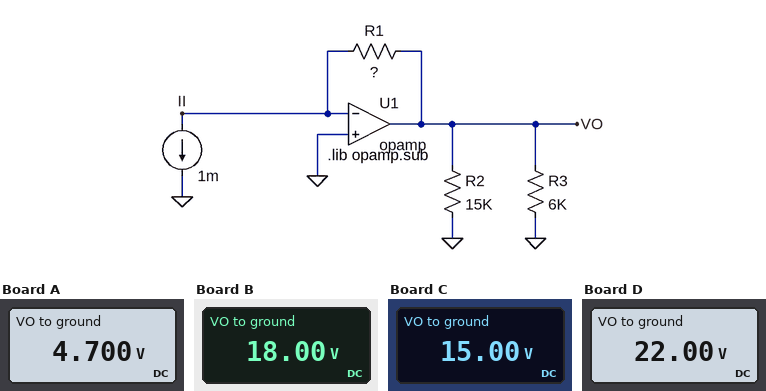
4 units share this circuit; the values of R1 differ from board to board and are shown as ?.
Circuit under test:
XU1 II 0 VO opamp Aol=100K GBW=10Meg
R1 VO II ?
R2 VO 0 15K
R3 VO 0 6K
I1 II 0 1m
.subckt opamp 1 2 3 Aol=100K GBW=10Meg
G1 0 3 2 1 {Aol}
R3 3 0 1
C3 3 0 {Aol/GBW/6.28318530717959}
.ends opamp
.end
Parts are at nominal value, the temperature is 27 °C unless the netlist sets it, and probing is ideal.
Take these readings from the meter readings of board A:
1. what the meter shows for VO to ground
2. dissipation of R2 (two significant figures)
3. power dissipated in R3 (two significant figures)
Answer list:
4.700 V
1.5 mW
3.7 mW
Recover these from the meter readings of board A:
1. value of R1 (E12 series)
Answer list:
4.7 kΩ
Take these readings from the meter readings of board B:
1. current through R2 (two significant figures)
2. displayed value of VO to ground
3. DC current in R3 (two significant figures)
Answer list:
1.2 mA
18.00 V
3.0 mA
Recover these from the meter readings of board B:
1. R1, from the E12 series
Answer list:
18 kΩ
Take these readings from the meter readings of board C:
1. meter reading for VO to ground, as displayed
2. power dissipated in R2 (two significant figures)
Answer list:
15.00 V
15 mW
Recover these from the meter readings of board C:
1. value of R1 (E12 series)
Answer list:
15 kΩ
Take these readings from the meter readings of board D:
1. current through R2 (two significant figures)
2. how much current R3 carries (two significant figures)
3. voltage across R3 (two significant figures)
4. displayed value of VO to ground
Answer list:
1.5 mA
3.7 mA
22 V
22.00 V
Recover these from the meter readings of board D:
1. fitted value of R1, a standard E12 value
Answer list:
22 kΩ
